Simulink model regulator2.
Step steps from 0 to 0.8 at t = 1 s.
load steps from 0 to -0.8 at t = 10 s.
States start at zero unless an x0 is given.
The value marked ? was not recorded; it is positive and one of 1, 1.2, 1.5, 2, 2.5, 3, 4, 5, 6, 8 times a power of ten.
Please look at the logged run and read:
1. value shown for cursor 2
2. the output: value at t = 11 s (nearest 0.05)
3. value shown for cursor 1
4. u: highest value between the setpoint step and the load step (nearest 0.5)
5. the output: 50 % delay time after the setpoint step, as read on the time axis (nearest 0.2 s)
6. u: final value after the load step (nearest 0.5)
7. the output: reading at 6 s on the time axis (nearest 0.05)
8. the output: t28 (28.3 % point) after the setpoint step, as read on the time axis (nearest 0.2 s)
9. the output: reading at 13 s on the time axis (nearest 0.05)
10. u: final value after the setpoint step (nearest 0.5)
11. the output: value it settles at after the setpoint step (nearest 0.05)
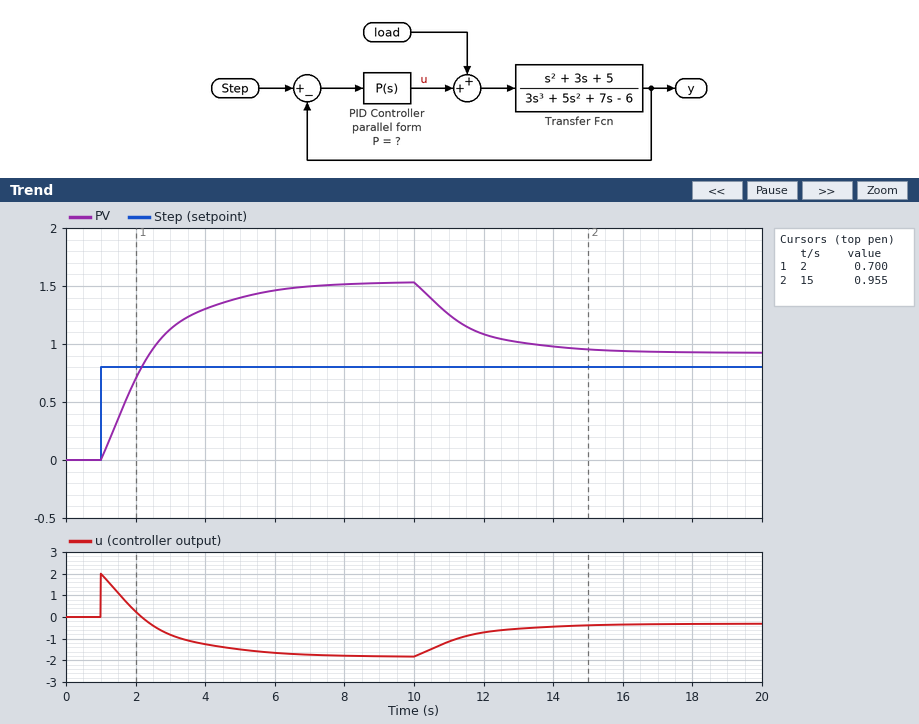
0.955
1.25
0.700
2.0
2.2 s
-0.5
1.45
1.6 s
1.00
-2.0
1.55
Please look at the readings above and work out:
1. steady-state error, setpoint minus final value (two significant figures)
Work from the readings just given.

-0.75
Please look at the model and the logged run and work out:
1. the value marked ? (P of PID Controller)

2.5
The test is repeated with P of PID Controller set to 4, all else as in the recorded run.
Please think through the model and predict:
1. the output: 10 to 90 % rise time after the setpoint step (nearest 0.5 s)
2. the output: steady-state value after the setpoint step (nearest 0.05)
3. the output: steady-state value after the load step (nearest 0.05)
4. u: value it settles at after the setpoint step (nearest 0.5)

1.5 s
1.15
0.85
-1.5
